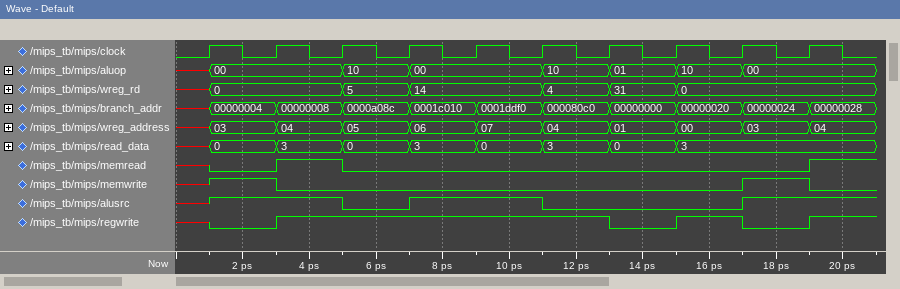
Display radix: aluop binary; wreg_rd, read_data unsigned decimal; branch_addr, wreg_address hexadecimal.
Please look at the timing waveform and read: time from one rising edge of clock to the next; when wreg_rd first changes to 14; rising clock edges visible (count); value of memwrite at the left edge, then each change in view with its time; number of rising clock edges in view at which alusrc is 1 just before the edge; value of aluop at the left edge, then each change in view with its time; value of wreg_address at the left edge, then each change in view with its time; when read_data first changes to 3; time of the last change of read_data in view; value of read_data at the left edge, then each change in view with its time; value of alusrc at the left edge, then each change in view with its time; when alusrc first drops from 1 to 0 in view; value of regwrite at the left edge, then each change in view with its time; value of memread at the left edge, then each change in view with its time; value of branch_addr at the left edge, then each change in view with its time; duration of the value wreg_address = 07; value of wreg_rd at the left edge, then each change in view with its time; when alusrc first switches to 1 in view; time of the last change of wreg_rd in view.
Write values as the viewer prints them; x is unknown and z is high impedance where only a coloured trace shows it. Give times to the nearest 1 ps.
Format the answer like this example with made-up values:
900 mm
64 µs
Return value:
2 ps
7 ps
10
x, 1 at 1 ps, 0 at 3 ps, 1 at 17 ps, 0 at 19 ps
5
x, 00 at 1 ps, 10 at 5 ps, 00 at 7 ps, 10 at 11 ps, 01 at 13 ps, 10 at 15 ps, 00 at 17 ps
x, 03 at 1 ps, 04 at 3 ps, 05 at 5 ps, 06 at 7 ps, 07 at 9 ps, 04 at 11 ps, 01 at 13 ps, 00 at 15 ps, 03 at 17 ps, 04 at 19 ps
3 ps
15 ps
x, 0 at 1 ps, 3 at 3 ps, 0 at 5 ps, 3 at 7 ps, 0 at 9 ps, 3 at 11 ps, 0 at 13 ps, 3 at 15 ps
x, 1 at 1 ps, 0 at 5 ps, 1 at 7 ps, 0 at 11 ps, 1 at 17 ps
5 ps
x, 0 at 1 ps, 1 at 3 ps, 0 at 13 ps, 1 at 15 ps, 0 at 17 ps, 1 at 19 ps
x, 0 at 1 ps, 1 at 3 ps, 0 at 5 ps, 1 at 19 ps
x, 00000004 at 1 ps, 00000008 at 3 ps, 0000a08c at 5 ps, 0001c010 at 7 ps, 0001ddf0 at 9 ps, 000080c0 at 11 ps, 00000000 at 13 ps, 00000020 at 15 ps, 00000024 at 17 ps, 00000028 at 19 ps
2 ps
x, 0 at 1 ps, 5 at 5 ps, 14 at 7 ps, 4 at 11 ps, 31 at 13 ps, 0 at 15 ps
1 ps
15 ps
